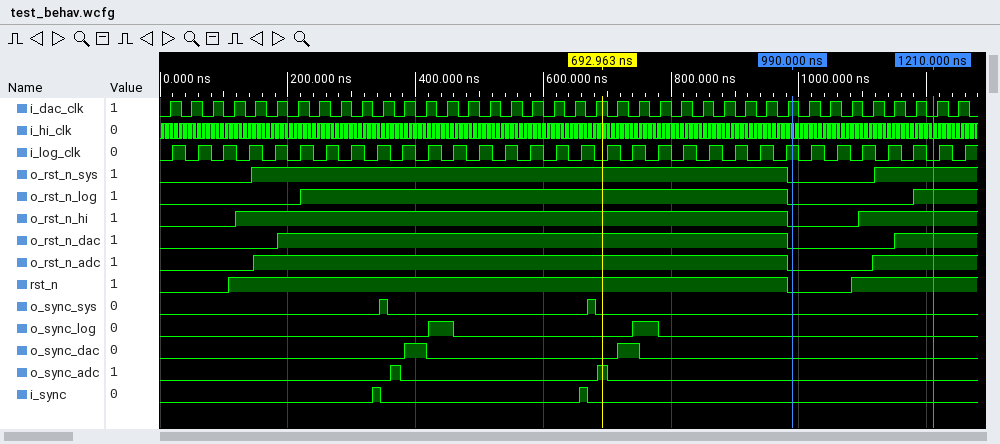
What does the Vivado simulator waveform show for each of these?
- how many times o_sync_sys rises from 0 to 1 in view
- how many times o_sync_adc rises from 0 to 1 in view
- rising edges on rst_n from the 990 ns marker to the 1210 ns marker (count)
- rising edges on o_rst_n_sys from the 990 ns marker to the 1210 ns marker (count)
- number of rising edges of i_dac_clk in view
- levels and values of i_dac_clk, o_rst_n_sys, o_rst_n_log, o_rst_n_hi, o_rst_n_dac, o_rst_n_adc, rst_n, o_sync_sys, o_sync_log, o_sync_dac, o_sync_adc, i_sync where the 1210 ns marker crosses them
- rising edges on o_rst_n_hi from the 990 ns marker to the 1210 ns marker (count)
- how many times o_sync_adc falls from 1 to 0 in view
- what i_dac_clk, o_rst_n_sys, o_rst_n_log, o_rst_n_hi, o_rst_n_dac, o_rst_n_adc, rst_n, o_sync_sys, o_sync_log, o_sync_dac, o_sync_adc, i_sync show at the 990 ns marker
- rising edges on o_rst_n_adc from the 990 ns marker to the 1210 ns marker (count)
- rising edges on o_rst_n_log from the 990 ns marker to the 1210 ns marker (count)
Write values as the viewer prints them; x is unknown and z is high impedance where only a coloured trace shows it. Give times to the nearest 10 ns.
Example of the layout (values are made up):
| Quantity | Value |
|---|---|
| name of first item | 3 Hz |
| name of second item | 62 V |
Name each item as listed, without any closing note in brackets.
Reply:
| Quantity | Value |
|---|---|
| how many times o_sync_sys rises from 0 to 1 in view | 2 |
| how many times o_sync_adc rises from 0 to 1 in view | 2 |
| rising edges on rst_n from the 990 ns marker to the 1210 ns marker | 1 |
| rising edges on o_rst_n_sys from the 990 ns marker to the 1210 ns marker | 1 |
| number of rising edges of i_dac_clk in view | 38 |
| levels and values of i_dac_clk, o_rst_n_sys, o_rst_n_log, o_rst_n_hi, o_rst_n_dac, o_rst_n_adc, rst_n, o_sync_sys, o_sync_log, o_sync_dac, o_sync_adc, i_sync where the 1210 ns marker crosses them | i_dac_clk=0, o_rst_n_sys=1, o_rst_n_log=1, o_rst_n_hi=1, o_rst_n_dac=1, o_rst_n_adc=1, rst_n=1, o_sync_sys=0, o_sync_log=0, o_sync_dac=0, o_sync_adc=0, i_sync=0 |
| rising edges on o_rst_n_hi from the 990 ns marker to the 1210 ns marker | 1 |
| how many times o_sync_adc falls from 1 to 0 in view | 2 |
| what i_dac_clk, o_rst_n_sys, o_rst_n_log, o_rst_n_hi, o_rst_n_dac, o_rst_n_adc, rst_n, o_sync_sys, o_sync_log, o_sync_dac, o_sync_adc, i_sync show at the 990 ns marker | i_dac_clk=1, o_rst_n_sys=0, o_rst_n_log=0, o_rst_n_hi=0, o_rst_n_dac=0, o_rst_n_adc=0, rst_n=0, o_sync_sys=0, o_sync_log=0, o_sync_dac=0, o_sync_adc=0, i_sync=0 |
| rising edges on o_rst_n_adc from the 990 ns marker to the 1210 ns marker | 1 |
| rising edges on o_rst_n_log from the 990 ns marker to the 1210 ns marker | 1 |
